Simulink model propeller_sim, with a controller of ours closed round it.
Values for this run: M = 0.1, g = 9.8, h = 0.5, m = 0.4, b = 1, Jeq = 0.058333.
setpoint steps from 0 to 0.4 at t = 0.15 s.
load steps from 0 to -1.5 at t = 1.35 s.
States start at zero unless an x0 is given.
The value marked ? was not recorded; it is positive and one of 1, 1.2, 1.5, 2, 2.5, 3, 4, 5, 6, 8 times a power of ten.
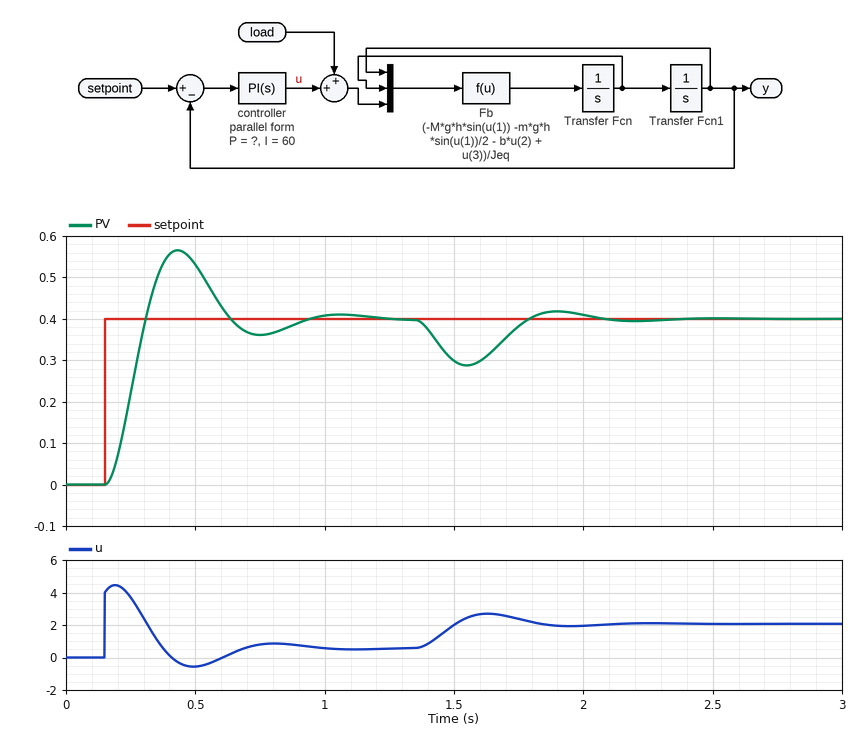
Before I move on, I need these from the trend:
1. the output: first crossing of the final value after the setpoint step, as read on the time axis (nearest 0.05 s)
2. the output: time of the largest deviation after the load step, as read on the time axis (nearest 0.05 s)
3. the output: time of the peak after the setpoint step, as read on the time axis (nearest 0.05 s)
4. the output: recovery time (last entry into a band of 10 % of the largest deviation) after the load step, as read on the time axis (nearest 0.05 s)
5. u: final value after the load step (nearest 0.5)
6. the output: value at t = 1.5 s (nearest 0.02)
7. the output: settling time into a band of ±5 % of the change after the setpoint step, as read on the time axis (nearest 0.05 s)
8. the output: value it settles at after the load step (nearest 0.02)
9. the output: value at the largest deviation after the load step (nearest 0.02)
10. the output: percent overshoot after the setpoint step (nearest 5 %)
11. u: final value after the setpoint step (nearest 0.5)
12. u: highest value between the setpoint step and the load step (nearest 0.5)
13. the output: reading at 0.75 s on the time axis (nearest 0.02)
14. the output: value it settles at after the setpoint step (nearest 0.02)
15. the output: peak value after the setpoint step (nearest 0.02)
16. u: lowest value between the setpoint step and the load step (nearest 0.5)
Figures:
0.30 s
1.55 s
0.45 s
2.00 s
2.0
0.30
0.85 s
0.40
0.28
40 %
0.5
4.5
0.36
0.40
0.56
-0.5
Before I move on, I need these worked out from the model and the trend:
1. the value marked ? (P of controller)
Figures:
10
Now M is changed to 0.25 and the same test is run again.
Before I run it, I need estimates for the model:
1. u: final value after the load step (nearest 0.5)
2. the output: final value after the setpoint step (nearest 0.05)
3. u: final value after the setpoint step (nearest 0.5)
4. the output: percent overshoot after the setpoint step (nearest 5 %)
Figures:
2.5
0.40
1.0
35 %
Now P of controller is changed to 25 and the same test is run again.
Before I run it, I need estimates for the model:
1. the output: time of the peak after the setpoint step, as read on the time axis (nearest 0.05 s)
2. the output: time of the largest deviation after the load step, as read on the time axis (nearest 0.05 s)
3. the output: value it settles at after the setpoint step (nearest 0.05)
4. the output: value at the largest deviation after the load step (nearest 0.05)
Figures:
0.30 s
1.50 s
0.40
0.35
